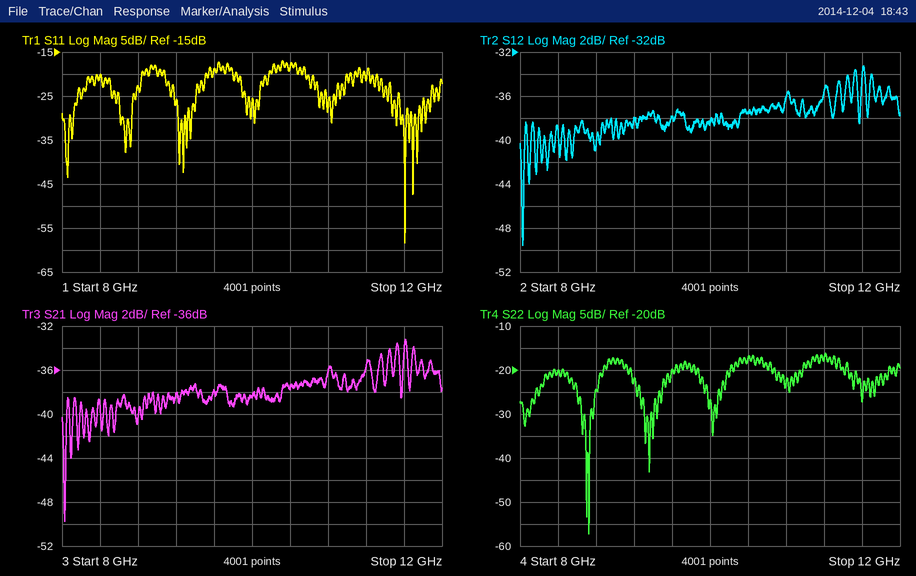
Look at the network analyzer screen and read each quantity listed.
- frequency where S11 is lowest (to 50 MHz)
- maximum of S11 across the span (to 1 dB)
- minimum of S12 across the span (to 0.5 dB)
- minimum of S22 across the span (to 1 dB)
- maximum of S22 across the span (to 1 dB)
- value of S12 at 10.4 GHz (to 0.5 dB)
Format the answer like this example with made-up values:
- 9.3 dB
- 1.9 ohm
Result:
- 11.60 GHz
- -17 dB
- -49.5 dB
- -57 dB
- -16 dB
- -37.5 dB
